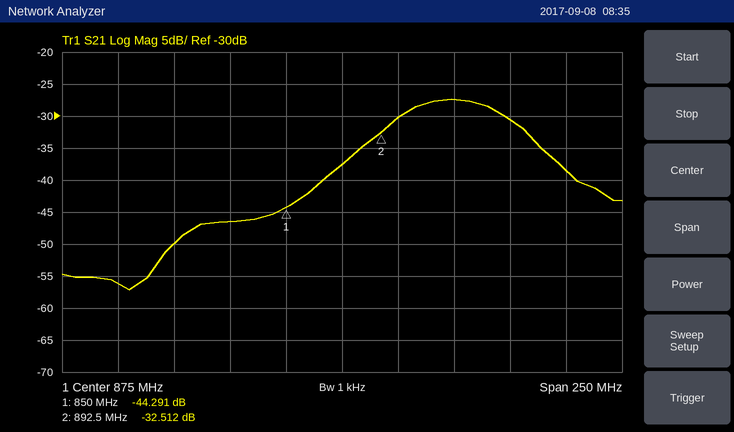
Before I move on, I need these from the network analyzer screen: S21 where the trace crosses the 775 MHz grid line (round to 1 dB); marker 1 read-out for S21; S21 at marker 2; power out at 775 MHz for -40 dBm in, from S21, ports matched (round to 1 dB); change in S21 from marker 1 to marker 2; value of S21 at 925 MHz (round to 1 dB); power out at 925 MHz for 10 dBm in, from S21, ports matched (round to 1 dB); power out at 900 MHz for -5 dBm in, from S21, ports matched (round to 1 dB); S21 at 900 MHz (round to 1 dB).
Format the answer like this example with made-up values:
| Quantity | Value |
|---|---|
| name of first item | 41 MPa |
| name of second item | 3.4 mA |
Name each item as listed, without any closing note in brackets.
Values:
| Quantity | Value |
|---|---|
| S21 where the trace crosses the 775 MHz grid line | -56 dB |
| marker 1 read-out for S21 | -44.291 dB |
| S21 at marker 2 | -32.512 dB |
| power out at 775 MHz for -40 dBm in, from S21, ports matched | -96 dBm |
| change in S21 from marker 1 to marker 2 | 11.779 dB |
| value of S21 at 925 MHz | -27 dB |
| power out at 925 MHz for 10 dBm in, from S21, ports matched | -17 dBm |
| power out at 900 MHz for -5 dBm in, from S21, ports matched | -35 dBm |
| S21 at 900 MHz | -30 dB |
